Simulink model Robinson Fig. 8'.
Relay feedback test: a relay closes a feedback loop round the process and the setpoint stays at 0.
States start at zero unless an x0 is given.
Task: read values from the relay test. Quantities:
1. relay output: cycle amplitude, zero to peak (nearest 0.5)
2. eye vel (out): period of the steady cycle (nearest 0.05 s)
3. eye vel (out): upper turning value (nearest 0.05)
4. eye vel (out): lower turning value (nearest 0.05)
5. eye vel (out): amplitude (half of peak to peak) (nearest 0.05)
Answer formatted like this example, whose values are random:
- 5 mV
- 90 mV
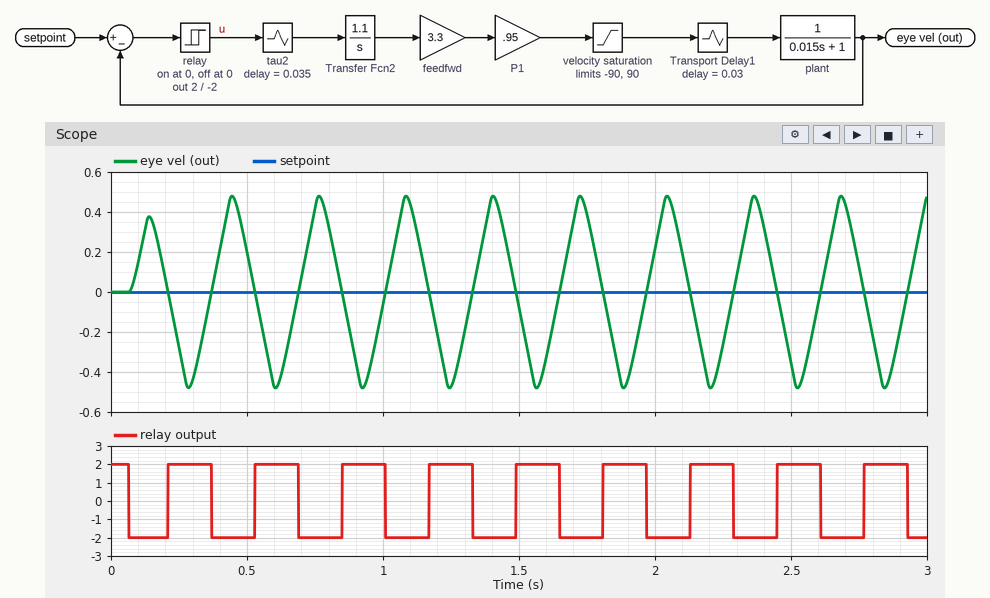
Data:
- 2.0
- 0.30 s
- 0.50
- -0.50
- 0.50
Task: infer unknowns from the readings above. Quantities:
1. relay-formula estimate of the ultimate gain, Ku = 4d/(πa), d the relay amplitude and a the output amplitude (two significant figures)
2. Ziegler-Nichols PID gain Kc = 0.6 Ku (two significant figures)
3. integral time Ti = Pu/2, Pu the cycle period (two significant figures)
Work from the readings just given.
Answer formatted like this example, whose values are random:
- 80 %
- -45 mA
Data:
- 5.1
- 3.1
- 0.15 s
